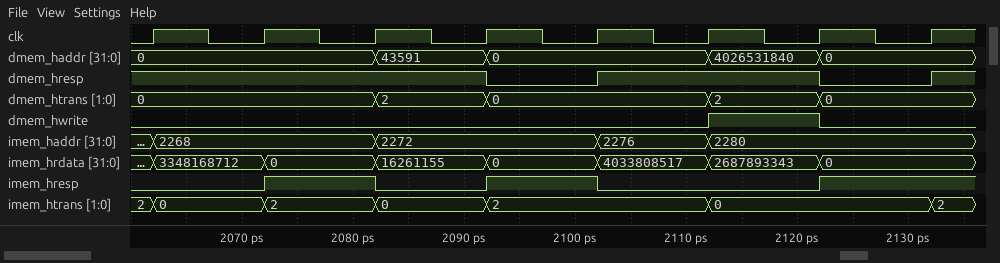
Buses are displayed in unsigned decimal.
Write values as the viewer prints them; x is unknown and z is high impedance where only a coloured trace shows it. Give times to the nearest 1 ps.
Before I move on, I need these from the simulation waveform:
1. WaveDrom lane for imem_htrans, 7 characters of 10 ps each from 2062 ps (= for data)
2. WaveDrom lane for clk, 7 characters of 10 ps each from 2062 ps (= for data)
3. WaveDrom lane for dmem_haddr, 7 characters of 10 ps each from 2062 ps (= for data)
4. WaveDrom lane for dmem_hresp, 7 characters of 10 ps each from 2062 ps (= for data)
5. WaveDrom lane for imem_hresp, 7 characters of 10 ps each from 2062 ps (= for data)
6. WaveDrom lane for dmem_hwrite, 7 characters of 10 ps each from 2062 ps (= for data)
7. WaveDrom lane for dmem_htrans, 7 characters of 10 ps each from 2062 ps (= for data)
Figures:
{name: 'imem_htrans', wave: '====.=.', data: '0 2 0 2 0'}
{name: 'clk', wave: 'p......'}
{name: 'dmem_haddr', wave: '=.==.==', data: '0 43591 0 4026531840 0'}
{name: 'dmem_hresp', wave: '1..01.0'}
{name: 'imem_hresp', wave: '01010.1'}
{name: 'dmem_hwrite', wave: '0....10'}
{name: 'dmem_htrans', wave: '=.==.==', data: '0 2 0 2 0'}
